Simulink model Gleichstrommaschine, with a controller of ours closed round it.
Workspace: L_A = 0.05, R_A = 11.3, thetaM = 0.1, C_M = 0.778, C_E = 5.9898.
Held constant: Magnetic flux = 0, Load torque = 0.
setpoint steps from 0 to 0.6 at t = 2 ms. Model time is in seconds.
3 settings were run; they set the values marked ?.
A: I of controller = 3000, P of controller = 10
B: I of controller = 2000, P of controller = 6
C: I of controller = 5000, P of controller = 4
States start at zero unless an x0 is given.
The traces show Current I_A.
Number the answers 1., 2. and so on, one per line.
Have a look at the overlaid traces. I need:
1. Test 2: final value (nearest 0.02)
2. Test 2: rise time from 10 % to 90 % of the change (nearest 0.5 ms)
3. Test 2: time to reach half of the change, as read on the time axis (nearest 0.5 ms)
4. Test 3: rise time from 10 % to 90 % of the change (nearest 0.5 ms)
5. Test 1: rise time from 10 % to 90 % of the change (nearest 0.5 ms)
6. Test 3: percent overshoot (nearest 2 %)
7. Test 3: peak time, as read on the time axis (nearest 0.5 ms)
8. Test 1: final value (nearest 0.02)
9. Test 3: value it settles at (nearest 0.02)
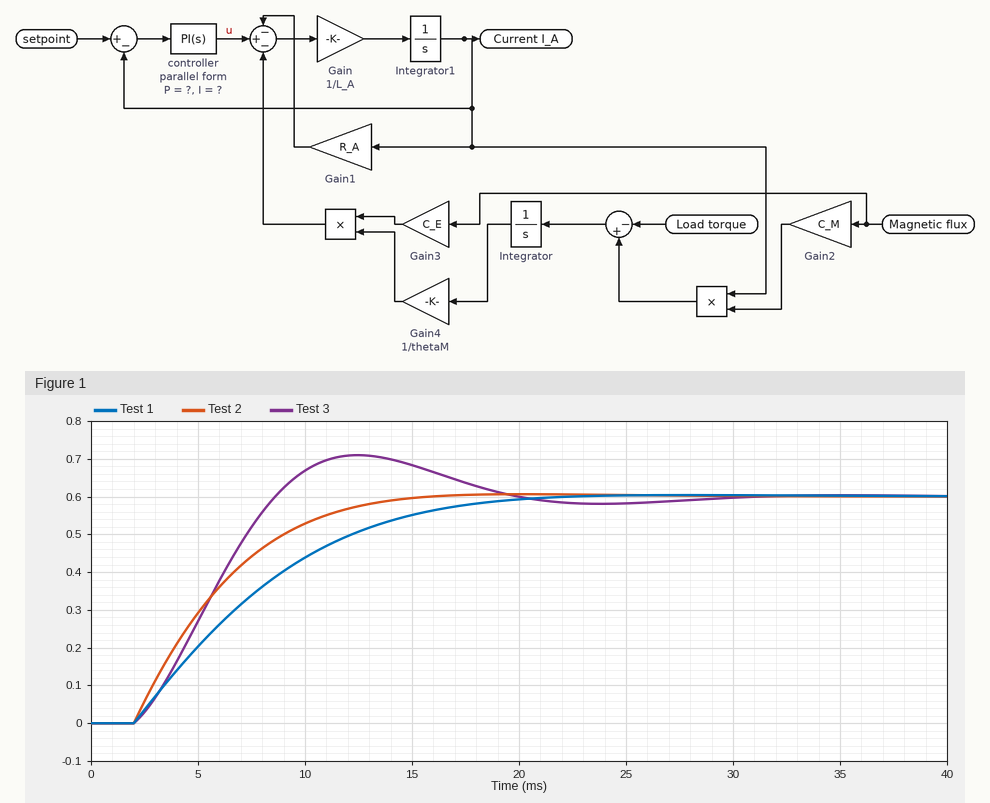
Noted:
1. 0.60
2. 8.0 ms
3. 5.0 ms
4. 5.0 ms
5. 11.5 ms
6. 18 %
7. 12.5 ms
8. 0.60
9. 0.60
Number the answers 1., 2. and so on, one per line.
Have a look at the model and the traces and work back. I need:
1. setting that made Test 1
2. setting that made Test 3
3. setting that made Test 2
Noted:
1. B
2. C
3. A
